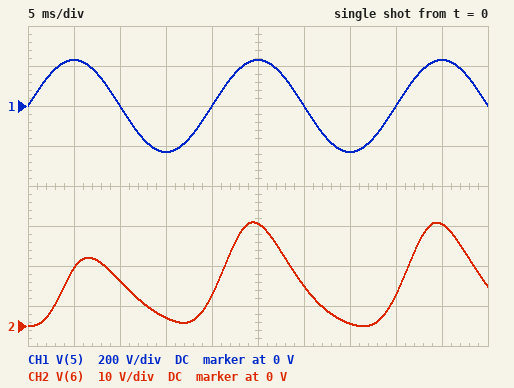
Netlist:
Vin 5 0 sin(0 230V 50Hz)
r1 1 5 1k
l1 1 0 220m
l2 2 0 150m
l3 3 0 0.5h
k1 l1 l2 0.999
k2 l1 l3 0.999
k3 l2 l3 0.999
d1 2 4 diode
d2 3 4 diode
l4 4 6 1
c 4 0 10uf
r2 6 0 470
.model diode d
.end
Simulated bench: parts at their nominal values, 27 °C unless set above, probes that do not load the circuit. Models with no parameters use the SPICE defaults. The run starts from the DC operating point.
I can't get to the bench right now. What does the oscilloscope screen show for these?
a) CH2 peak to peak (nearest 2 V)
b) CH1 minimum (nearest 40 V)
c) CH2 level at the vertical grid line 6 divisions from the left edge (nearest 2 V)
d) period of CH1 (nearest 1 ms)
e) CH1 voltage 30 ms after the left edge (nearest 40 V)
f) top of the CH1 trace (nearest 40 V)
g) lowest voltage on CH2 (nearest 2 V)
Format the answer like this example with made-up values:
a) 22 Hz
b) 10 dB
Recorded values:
a) 26 V
b) -240 V
c) 10 V
d) 20 ms
e) 0 V
f) 240 V
g) 0 V
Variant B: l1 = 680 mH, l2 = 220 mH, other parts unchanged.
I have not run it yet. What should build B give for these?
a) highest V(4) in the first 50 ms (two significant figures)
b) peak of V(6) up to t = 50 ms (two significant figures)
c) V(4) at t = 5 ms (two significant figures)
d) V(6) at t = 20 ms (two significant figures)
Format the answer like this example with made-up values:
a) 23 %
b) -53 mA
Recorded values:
a) 49 V
b) 41 V
c) 34 V
d) 12 V
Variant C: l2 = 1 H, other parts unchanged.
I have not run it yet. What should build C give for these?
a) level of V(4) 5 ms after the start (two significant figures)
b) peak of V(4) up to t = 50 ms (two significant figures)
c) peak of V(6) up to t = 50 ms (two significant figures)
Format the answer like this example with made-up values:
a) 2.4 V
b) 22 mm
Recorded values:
a) 21 V
b) 37 V
c) 32 V
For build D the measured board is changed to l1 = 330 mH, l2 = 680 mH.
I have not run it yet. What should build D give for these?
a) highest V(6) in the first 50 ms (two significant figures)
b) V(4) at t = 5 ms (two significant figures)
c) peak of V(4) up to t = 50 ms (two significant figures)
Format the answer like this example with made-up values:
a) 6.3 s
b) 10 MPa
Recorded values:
a) 35 V
b) 27 V
c) 41 V
